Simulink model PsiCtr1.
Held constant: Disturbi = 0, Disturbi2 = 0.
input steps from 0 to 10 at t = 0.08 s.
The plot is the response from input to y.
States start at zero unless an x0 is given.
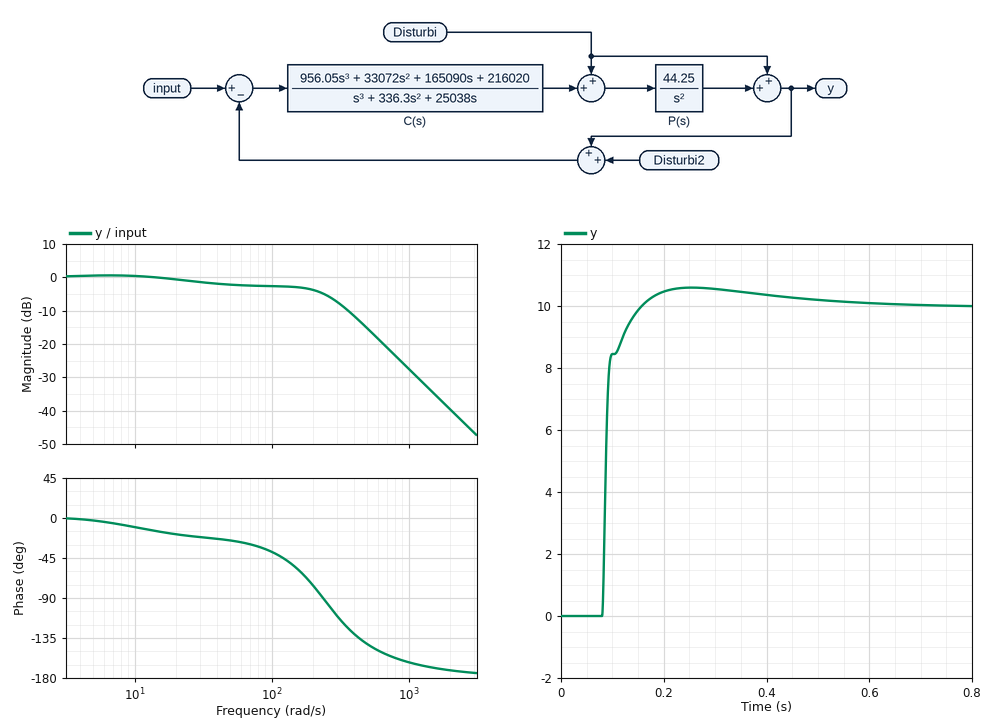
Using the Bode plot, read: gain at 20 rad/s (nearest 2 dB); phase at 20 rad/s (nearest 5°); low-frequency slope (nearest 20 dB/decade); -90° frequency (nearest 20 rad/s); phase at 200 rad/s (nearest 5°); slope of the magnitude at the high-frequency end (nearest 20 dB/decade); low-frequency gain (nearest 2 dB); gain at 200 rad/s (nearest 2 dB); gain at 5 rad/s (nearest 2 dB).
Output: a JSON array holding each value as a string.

["0 dB", "-20°", "0 dB/decade", "240 rad/s", "-75°", "-40 dB/decade", "0 dB", "-4 dB", "0 dB"]
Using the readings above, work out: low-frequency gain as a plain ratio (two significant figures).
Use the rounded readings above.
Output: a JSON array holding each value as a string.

["1.0"]
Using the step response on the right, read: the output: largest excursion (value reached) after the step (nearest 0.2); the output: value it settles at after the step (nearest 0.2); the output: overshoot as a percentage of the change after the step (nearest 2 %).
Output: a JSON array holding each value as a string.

["10.6", "10.0", "6 %"]
